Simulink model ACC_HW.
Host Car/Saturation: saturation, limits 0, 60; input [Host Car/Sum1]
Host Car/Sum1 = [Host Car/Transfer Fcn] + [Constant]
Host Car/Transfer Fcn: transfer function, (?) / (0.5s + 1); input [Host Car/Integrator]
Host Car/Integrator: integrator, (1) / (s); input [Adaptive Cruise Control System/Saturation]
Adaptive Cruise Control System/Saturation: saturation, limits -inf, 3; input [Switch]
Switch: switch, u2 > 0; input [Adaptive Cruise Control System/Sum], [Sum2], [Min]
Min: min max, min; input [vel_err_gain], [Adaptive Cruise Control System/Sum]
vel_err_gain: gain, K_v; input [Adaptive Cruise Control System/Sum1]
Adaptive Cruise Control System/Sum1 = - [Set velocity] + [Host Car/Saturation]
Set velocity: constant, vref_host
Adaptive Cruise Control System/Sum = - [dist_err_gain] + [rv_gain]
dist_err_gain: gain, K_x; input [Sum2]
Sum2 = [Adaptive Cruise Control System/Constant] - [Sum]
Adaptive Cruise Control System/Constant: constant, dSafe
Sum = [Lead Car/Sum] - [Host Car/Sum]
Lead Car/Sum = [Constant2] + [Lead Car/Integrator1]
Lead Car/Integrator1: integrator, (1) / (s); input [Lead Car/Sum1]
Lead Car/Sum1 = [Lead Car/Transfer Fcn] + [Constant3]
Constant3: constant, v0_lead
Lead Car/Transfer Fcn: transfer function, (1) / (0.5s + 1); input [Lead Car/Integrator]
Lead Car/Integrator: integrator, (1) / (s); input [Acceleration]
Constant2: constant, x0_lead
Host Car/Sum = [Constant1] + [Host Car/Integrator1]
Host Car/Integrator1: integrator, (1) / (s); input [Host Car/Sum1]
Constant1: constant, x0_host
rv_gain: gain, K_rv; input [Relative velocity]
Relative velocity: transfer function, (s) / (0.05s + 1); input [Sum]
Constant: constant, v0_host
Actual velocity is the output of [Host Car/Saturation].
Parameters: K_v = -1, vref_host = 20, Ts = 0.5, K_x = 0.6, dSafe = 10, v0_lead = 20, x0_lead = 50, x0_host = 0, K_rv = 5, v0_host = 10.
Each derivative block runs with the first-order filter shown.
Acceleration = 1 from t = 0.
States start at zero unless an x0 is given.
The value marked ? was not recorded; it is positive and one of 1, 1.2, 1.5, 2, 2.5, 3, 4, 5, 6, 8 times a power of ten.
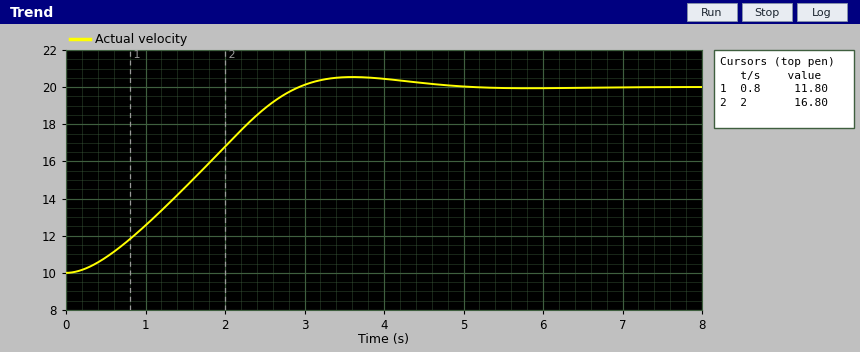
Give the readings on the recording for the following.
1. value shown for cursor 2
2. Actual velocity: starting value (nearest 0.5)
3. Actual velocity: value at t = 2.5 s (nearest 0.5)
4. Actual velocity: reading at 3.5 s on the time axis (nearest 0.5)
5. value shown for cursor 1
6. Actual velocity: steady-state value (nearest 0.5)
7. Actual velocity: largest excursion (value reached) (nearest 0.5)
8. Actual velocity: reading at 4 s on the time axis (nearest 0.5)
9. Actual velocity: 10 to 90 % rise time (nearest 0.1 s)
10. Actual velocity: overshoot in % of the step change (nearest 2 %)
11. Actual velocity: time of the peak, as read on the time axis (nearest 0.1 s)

16.80
10.0
19.0
20.5
11.80
20.0
20.5
20.5
2.0 s
6 %
3.6 s
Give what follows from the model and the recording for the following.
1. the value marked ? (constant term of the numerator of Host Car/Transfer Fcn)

1.5
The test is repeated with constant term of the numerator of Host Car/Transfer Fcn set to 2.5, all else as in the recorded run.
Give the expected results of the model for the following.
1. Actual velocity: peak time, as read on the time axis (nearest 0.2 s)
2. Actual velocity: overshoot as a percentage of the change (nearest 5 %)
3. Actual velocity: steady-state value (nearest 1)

2.4 s
10 %
20
